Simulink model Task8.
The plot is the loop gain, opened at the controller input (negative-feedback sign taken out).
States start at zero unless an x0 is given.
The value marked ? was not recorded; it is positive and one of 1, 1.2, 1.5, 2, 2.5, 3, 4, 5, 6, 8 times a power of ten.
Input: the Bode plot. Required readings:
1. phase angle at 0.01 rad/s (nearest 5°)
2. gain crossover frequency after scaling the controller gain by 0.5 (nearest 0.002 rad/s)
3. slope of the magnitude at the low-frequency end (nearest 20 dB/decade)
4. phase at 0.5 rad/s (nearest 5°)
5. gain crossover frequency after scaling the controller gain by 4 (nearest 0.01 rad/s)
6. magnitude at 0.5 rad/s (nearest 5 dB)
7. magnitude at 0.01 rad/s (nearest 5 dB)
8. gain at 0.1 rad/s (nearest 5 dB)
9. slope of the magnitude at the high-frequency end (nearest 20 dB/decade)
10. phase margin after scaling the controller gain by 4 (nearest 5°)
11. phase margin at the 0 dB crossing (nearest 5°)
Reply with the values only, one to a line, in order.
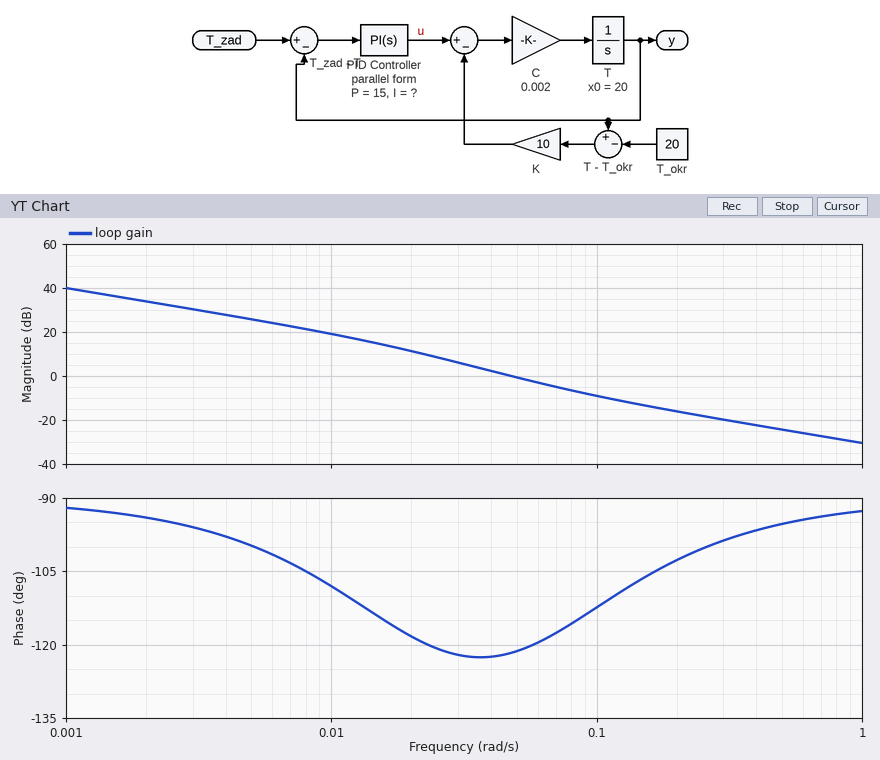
-110°
0.030 rad/s
-20 dB/decade
-95°
0.13 rad/s
-25 dB
20 dB
-10 dB
-20 dB/decade
70°
60°
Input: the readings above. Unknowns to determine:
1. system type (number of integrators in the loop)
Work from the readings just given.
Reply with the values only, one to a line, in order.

1
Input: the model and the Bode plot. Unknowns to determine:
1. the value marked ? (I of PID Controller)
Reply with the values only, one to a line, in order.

1
